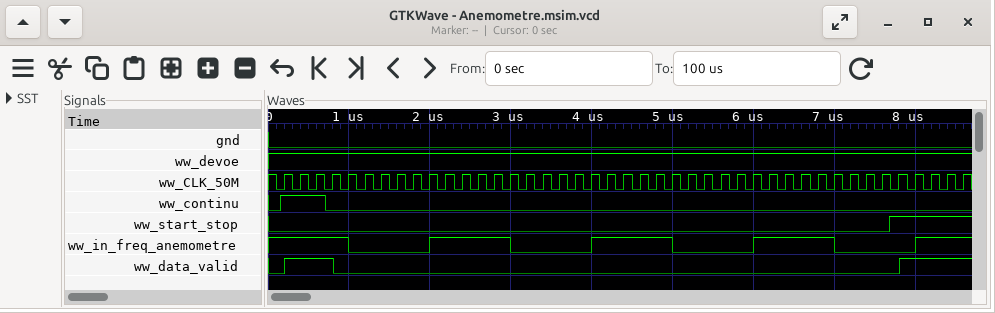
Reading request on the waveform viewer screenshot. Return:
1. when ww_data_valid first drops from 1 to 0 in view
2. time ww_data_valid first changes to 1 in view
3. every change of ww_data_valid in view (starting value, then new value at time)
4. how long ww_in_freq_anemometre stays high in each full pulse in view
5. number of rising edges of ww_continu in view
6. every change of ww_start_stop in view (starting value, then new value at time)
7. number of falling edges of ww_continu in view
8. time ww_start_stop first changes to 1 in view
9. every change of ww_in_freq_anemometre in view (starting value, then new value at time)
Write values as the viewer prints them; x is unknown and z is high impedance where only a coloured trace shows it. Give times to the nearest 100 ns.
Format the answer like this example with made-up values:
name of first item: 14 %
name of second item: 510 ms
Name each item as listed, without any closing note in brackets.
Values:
when ww_data_valid first drops from 1 to 0 in view: 800 ns
time ww_data_valid first changes to 1 in view: 200 ns
every change of ww_data_valid in view: 0, 1 at 200 ns, 0 at 800 ns, 1 at 7800 ns
how long ww_in_freq_anemometre stays high in each full pulse in view: 1000 ns, 1000 ns, 1000 ns
number of rising edges of ww_continu in view: 1
every change of ww_start_stop in view: 0, 1 at 7700 ns
number of falling edges of ww_continu in view: 1
time ww_start_stop first changes to 1 in view: 7700 ns
every change of ww_in_freq_anemometre in view: 1, 0 at 1000 ns, 1 at 2000 ns, 0 at 3000 ns, 1 at 4000 ns, 0 at 5000 ns, 1 at 6000 ns, 0 at 7000 ns, 1 at 8000 ns
